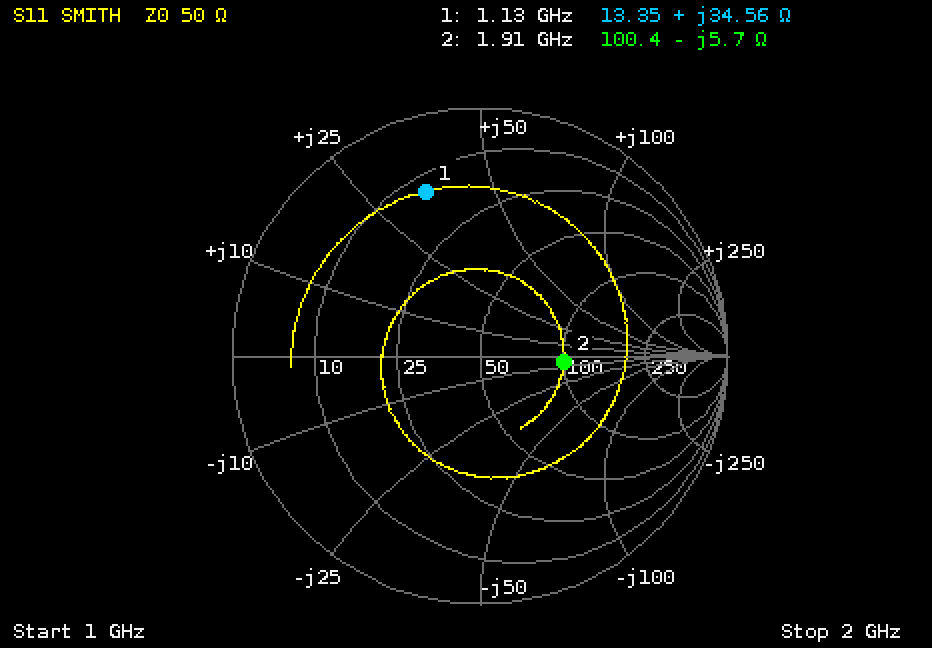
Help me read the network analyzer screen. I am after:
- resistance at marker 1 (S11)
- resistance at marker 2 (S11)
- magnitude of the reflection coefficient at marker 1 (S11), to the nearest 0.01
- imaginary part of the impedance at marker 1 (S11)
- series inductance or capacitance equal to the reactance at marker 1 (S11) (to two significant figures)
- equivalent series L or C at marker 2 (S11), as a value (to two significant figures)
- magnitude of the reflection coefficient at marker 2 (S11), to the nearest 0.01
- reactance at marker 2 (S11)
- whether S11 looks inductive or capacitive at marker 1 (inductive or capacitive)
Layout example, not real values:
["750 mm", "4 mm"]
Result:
["13.35 Ω", "100.4 Ω", "0.70", "+34.56 Ω", "4.9 nH", "15 pF", "0.34", "-5.7 Ω", "inductive"]
